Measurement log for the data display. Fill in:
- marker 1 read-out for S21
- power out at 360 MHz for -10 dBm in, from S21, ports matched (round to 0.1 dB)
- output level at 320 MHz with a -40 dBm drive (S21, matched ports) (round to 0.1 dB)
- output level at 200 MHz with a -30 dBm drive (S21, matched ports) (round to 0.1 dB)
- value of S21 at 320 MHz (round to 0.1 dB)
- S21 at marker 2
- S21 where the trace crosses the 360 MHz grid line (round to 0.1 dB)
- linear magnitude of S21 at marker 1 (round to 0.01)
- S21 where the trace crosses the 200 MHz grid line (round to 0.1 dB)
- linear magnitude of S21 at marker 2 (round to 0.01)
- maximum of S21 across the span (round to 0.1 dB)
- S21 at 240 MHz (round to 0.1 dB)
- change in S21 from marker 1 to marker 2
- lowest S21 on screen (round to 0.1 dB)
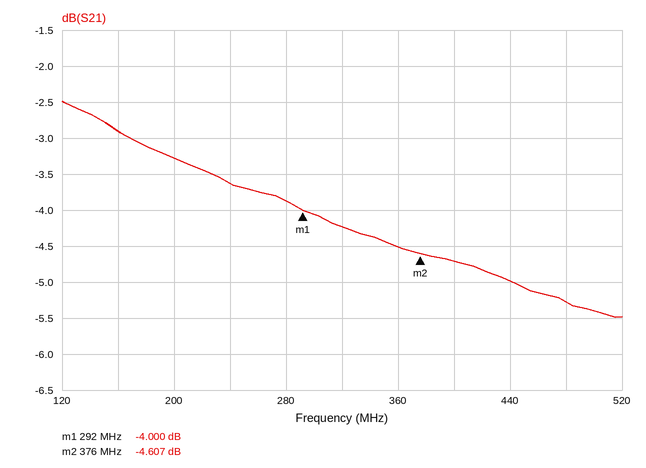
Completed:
-4.000 dB
-14.5 dBm
-44.2 dBm
-33.3 dBm
-4.2 dB
-4.607 dB
-4.5 dB
0.63
-3.3 dB
0.59
-2.5 dB
-3.6 dB
-0.607 dB
-5.5 dB
